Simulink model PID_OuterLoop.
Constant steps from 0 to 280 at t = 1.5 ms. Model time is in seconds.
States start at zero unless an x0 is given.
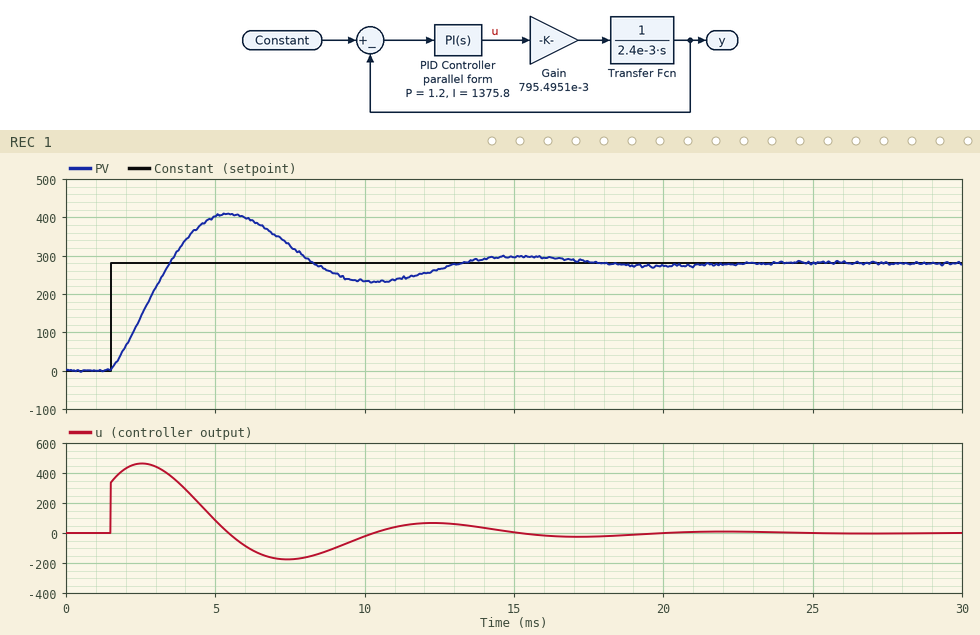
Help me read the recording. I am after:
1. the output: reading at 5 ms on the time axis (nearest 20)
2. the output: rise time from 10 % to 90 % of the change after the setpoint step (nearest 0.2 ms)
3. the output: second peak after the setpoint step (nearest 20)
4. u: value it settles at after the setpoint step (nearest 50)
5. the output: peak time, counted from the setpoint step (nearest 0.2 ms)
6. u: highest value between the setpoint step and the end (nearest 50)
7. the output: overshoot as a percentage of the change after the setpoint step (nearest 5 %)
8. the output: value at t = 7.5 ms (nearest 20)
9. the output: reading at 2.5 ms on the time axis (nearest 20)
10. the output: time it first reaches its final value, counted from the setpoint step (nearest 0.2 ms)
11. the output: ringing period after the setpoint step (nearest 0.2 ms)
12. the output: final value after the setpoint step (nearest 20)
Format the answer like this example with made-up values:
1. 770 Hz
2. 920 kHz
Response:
1. 400
2. 1.6 ms
3. 300
4. 0
5. 4.0 ms
6. 450
7. 45 %
8. 320
9. 140
10. 2.0 ms
11. 9.8 ms
12. 280
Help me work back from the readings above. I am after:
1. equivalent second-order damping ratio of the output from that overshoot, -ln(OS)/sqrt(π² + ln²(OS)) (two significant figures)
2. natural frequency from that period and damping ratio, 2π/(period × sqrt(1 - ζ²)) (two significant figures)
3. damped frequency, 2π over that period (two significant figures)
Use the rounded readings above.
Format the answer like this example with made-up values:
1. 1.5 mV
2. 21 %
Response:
1. 0.25
2. 0.66 rad/ms
3. 0.64 rad/ms
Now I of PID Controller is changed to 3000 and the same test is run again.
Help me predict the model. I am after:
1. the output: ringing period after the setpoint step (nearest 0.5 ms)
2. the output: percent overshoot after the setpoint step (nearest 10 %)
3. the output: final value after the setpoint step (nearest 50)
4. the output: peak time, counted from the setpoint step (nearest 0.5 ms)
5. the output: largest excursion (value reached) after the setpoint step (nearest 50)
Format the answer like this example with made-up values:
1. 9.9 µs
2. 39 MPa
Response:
1. 6.5 ms
2. 60 %
3. 300
4. 3.0 ms
5. 450
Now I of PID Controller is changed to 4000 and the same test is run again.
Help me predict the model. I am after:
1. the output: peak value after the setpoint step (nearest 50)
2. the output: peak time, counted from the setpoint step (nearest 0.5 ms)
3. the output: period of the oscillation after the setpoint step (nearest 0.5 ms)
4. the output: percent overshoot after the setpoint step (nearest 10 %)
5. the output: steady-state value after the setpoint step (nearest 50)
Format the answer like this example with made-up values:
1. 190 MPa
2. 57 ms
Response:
1. 450
2. 2.5 ms
3. 5.5 ms
4. 60 %
5. 300
